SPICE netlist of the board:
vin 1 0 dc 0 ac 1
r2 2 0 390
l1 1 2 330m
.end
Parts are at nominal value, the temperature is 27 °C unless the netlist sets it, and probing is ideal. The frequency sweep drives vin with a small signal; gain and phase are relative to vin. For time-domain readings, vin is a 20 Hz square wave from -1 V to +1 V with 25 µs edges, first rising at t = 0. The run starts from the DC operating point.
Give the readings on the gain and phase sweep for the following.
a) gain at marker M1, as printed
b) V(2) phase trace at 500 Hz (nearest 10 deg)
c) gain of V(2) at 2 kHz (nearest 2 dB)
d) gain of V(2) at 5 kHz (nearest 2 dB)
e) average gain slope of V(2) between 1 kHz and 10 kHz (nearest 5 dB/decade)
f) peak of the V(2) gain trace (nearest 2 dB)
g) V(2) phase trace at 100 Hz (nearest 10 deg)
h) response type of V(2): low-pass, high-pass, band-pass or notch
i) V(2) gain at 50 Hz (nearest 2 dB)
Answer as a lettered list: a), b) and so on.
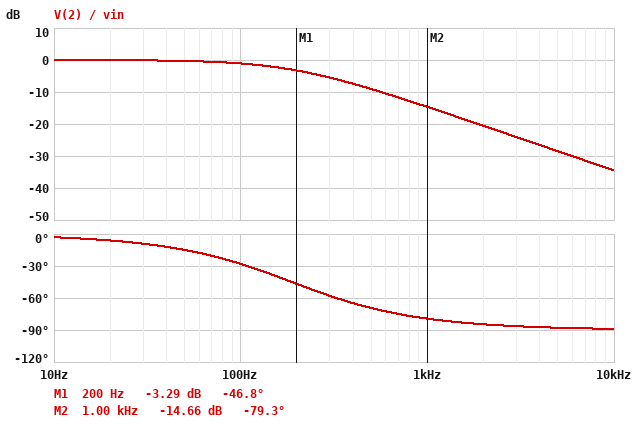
a) -3.29 dB
b) -70 deg
c) -20 dB
d) -28 dB
e) -20 dB/decade
f) 0 dB
g) -30 deg
h) low-pass
i) 0 dB
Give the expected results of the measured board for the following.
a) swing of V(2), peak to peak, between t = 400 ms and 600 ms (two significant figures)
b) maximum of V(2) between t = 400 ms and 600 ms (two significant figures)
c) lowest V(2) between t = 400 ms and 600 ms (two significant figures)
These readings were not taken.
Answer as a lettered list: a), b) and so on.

a) 2.0 V
b) 1.0 V
c) -1.0 V
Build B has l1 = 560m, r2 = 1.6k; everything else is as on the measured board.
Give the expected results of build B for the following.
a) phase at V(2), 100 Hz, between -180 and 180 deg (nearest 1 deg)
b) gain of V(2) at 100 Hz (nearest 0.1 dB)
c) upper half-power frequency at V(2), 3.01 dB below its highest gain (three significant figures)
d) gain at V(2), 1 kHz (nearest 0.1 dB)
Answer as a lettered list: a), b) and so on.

a) -12 deg
b) -0.2 dB
c) 455 Hz
d) -7.7 dB
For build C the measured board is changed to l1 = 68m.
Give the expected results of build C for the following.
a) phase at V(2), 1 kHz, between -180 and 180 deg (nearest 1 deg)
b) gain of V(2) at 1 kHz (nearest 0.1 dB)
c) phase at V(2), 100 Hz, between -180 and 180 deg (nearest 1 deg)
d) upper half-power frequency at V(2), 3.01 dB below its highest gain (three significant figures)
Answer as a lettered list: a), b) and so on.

a) -48 deg
b) -3.4 dB
c) -6 deg
d) 913 Hz
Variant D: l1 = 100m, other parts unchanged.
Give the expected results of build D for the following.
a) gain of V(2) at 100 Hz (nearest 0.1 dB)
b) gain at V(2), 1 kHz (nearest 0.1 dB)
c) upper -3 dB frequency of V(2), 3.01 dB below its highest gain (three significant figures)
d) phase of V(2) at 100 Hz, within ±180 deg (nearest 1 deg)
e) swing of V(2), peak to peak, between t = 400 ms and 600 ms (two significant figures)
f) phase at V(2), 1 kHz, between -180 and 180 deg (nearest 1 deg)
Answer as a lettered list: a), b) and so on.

a) -0.1 dB
b) -5.6 dB
c) 621 Hz
d) -9 deg
e) 2.0 V
f) -58 deg
